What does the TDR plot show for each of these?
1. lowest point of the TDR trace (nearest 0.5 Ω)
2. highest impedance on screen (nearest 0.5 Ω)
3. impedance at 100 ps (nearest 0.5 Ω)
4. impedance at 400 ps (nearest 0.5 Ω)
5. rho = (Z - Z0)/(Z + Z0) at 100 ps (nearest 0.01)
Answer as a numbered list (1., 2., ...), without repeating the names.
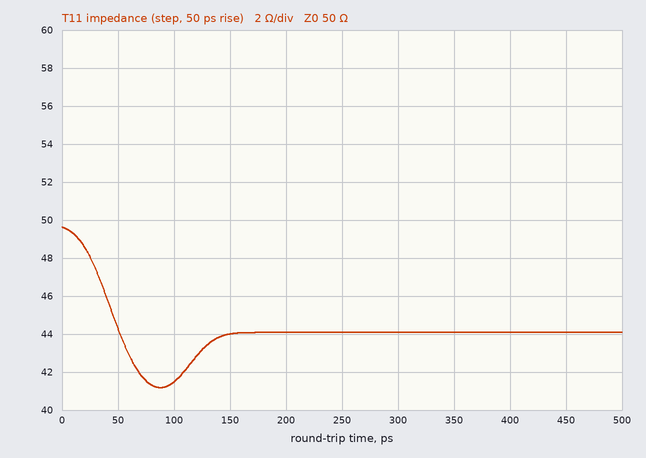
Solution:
1. 41.0 Ω
2. 49.5 Ω
3. 41.5 Ω
4. 44.0 Ω
5. -0.09
